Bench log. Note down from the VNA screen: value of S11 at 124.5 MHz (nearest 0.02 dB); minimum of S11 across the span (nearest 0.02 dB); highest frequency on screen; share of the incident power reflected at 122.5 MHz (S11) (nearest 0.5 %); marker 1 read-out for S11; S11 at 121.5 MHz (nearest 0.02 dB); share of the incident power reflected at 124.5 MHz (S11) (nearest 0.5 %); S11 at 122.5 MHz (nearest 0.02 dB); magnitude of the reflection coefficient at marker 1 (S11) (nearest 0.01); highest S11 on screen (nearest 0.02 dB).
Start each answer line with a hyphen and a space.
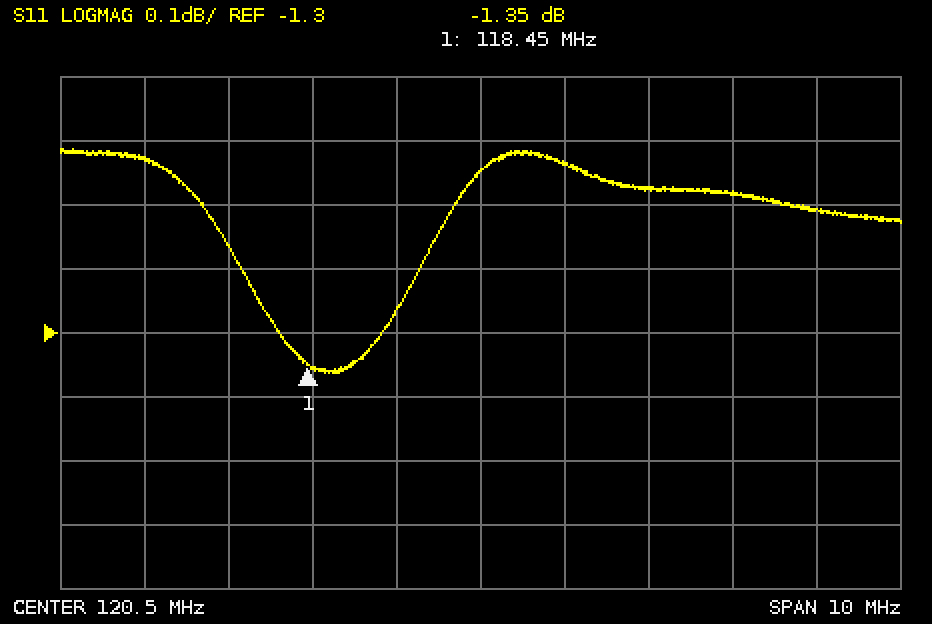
- -1.10 dB
- -1.36 dB
- 125.5 MHz
- 78.0 %
- -1.35 dB
- -1.04 dB
- 77.5 %
- -1.08 dB
- 0.86
- -1.02 dB
